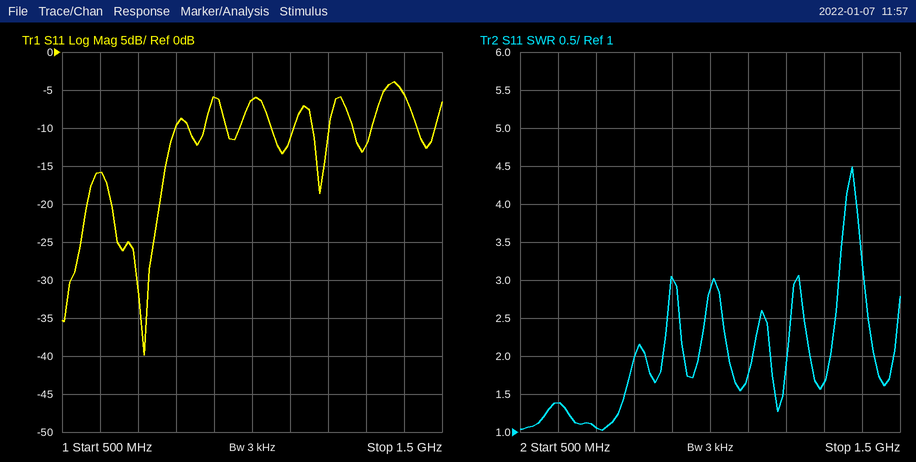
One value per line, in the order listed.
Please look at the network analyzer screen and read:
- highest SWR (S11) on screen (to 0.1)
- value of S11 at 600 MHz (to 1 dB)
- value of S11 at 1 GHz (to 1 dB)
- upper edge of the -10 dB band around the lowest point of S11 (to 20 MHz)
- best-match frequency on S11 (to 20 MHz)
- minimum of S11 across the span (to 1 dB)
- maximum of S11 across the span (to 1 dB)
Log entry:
4.5
-16 dB
-6 dB
800 MHz
720 MHz
-40 dB
-4 dB
